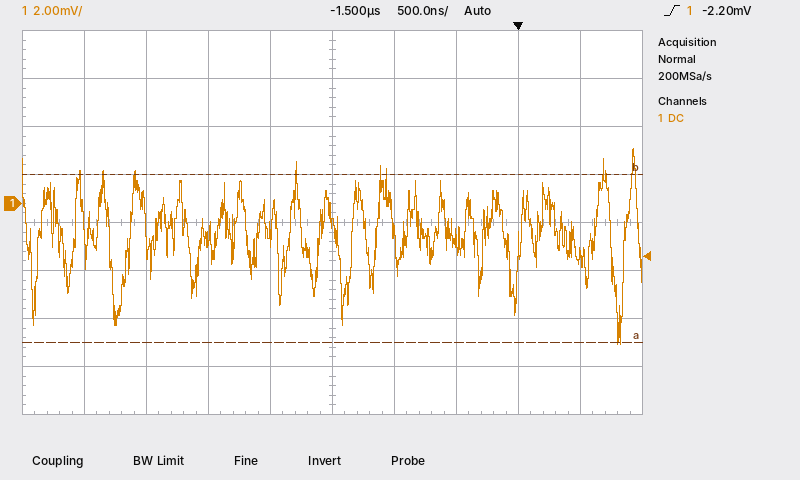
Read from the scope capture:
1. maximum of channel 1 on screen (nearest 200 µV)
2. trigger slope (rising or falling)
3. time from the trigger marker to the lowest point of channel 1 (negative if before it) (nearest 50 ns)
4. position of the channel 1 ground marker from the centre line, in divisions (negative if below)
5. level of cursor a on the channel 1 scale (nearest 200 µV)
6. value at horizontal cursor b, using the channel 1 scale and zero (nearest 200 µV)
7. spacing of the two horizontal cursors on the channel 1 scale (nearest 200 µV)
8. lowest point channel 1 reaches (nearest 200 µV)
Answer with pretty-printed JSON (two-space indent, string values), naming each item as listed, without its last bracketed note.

{
  "maximum of channel 1 on screen": "2.2 mV",
  "trigger slope": "rising",
  "time from the trigger marker to the lowest point of channel 1 (negative if before it)": "+800 ns",
  "position of the channel 1 ground marker from the centre line, in divisions": "+0.4 div",
  "level of cursor a on the channel 1 scale": "-5.8 mV",
  "value at horizontal cursor b, using the channel 1 scale and zero": "1.2 mV",
  "spacing of the two horizontal cursors on the channel 1 scale": "7.0 mV",
  "lowest point channel 1 reaches": "-5.8 mV"
}
